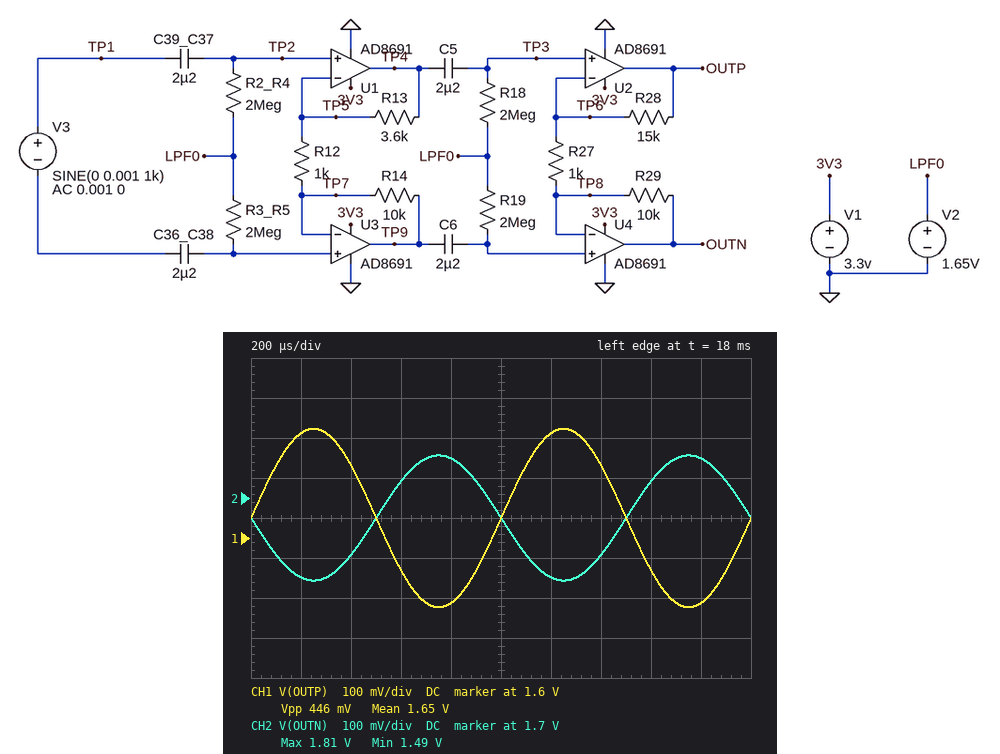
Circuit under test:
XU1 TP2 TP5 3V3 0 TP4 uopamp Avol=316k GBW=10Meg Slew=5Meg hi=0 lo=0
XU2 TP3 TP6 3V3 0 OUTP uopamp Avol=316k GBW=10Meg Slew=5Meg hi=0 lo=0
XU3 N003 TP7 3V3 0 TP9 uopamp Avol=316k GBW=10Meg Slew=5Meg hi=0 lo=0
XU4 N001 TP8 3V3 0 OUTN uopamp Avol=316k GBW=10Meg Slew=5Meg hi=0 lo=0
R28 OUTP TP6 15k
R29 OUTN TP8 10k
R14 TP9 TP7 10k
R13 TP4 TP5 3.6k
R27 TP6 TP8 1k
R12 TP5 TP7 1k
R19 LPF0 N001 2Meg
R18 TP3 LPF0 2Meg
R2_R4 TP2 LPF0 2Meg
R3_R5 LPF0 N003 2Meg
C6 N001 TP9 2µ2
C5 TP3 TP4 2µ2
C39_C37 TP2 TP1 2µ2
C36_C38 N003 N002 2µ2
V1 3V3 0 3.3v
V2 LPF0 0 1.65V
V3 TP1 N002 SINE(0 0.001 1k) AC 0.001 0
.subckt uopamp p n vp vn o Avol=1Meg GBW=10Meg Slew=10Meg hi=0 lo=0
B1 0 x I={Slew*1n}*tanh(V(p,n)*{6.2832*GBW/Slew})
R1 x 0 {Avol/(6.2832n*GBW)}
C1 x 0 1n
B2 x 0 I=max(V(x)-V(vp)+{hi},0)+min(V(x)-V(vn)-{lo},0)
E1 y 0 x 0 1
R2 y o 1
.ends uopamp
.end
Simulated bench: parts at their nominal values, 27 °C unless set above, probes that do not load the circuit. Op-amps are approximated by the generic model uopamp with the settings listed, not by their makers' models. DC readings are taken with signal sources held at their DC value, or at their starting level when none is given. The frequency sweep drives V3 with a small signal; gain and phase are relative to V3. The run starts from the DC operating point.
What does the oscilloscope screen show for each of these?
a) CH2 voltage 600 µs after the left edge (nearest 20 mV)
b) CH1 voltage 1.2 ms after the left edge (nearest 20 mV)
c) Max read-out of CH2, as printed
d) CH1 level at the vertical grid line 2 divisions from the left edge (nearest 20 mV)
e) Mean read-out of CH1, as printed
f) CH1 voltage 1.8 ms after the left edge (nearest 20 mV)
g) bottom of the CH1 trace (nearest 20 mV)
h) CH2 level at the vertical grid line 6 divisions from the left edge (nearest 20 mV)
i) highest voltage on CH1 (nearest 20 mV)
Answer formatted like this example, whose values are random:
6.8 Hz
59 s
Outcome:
1.74 V
1.86 V
1.81 V
1.78 V
1.65 V
1.44 V
1.42 V
1.50 V
1.88 V
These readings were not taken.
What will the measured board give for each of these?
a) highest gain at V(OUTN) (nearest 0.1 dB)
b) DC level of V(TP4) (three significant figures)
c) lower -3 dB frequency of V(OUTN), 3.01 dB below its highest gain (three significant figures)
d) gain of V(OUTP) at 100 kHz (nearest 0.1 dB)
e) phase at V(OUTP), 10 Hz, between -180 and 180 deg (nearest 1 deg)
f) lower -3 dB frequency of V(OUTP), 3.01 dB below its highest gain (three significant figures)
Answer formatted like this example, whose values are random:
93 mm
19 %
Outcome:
43.9 dB
1.65 V
56.2 mHz
46.6 dB
0 deg
56.2 mHz
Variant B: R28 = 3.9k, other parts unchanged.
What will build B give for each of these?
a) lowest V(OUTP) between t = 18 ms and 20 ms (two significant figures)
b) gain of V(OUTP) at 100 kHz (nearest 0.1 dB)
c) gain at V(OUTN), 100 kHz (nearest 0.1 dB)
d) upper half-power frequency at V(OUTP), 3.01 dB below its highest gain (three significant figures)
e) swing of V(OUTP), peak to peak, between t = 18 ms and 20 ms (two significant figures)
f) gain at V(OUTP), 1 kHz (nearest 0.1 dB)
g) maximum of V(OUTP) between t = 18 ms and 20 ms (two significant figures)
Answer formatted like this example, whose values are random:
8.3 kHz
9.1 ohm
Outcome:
1.6 V
35.5 dB
43.7 dB
435 kHz
120 mV
35.7 dB
1.7 V
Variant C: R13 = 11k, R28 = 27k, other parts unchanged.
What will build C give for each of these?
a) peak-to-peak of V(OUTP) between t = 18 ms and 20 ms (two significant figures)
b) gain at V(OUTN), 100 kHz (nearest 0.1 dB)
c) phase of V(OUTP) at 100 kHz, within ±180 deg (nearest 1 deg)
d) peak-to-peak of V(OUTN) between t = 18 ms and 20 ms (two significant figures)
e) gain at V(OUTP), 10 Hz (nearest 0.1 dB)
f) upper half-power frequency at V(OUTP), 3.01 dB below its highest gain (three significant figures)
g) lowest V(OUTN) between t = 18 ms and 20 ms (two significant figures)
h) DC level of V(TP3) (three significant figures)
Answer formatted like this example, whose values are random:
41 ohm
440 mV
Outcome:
1.2 V
46.5 dB
-33 deg
460 mV
55.6 dB
211 kHz
1.4 V
1.65 V
